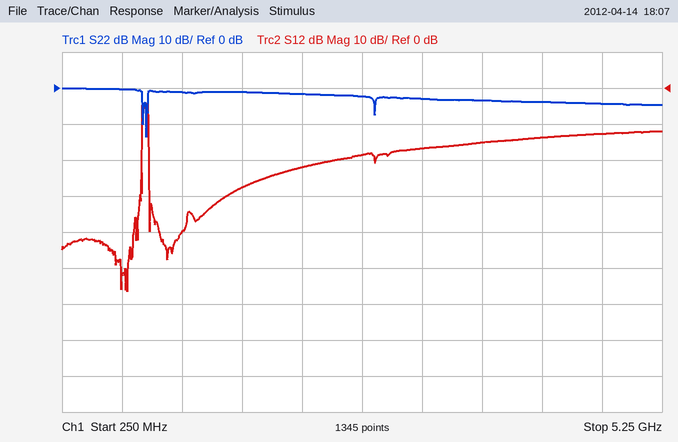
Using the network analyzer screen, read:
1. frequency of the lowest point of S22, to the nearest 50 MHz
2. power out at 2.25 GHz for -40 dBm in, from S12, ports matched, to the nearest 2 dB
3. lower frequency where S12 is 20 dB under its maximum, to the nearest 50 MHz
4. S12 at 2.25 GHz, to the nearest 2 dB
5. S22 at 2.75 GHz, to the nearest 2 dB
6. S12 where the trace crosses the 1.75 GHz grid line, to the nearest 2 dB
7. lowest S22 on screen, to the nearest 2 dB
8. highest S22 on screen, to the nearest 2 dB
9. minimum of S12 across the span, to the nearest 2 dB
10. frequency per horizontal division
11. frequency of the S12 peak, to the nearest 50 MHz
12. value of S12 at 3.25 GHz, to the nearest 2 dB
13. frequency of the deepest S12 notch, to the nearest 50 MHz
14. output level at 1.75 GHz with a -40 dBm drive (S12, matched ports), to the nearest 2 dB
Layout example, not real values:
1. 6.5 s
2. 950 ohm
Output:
1. 950 MHz
2. -62 dBm
3. 900 MHz
4. -22 dB
5. -2 dB
6. -28 dB
7. -14 dB
8. 0 dB
9. -56 dB
10. 500 MHz
11. 950 MHz
12. -16 dB
13. 800 MHz
14. -68 dBm
